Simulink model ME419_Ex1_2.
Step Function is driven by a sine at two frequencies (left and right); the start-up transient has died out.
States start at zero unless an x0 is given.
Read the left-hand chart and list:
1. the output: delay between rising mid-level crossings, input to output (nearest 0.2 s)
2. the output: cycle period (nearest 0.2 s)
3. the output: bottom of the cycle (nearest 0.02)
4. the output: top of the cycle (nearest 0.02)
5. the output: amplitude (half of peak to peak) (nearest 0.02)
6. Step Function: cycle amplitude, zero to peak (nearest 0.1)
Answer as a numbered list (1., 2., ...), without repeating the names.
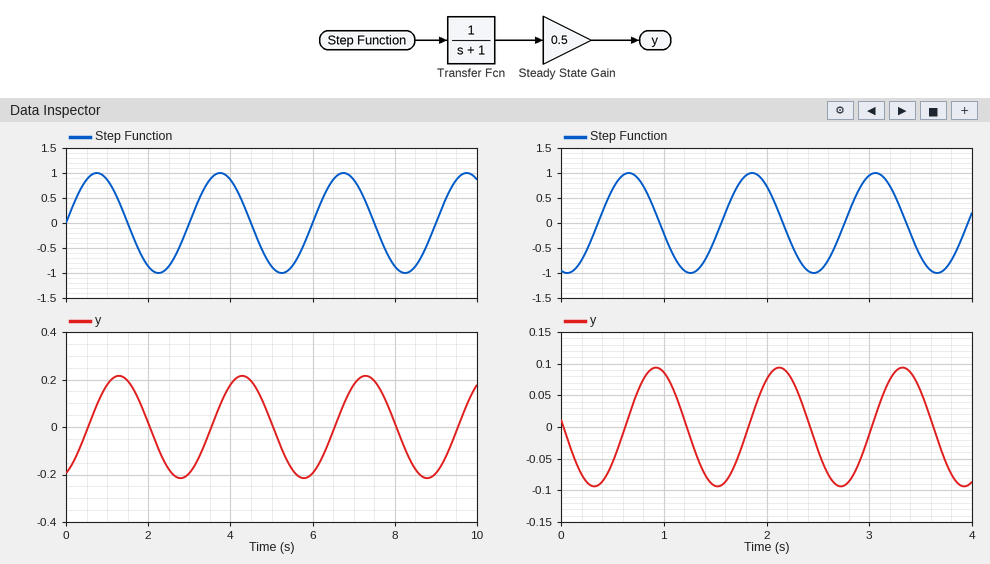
1. 0.6 s
2. 3.0 s
3. -0.22
4. 0.22
5. 0.22
6. 1.0
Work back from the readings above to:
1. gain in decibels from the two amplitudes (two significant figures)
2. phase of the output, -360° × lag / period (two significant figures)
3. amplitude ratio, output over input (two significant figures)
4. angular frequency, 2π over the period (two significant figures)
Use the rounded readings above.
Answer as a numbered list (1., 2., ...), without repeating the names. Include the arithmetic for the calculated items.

1. 20 log10(0.22 / 1) = -13 dB
2. -360 × 0.6 / 3 = -72°
3. 0.22 / 1 = 0.22
4. 2π / 3 = 2.1 rad/s
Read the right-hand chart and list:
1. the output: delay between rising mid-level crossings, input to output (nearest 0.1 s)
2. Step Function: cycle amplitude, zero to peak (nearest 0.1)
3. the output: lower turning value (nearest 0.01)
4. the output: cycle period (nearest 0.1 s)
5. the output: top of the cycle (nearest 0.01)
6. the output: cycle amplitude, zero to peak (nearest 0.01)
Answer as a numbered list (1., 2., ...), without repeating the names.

1. 0.3 s
2. 1.0
3. -0.09
4. 1.2 s
5. 0.09
6. 0.09
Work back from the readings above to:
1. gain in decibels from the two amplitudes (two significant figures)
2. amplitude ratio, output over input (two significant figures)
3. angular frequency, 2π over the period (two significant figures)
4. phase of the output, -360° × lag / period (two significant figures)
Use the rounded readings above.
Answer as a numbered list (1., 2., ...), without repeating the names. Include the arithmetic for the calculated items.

1. 20 log10(0.09 / 1) = -21 dB
2. 0.09 / 1 = 0.090
3. 2π / 1.2 = 5.2 rad/s
4. -360 × 0.3 / 1.2 = -90°
